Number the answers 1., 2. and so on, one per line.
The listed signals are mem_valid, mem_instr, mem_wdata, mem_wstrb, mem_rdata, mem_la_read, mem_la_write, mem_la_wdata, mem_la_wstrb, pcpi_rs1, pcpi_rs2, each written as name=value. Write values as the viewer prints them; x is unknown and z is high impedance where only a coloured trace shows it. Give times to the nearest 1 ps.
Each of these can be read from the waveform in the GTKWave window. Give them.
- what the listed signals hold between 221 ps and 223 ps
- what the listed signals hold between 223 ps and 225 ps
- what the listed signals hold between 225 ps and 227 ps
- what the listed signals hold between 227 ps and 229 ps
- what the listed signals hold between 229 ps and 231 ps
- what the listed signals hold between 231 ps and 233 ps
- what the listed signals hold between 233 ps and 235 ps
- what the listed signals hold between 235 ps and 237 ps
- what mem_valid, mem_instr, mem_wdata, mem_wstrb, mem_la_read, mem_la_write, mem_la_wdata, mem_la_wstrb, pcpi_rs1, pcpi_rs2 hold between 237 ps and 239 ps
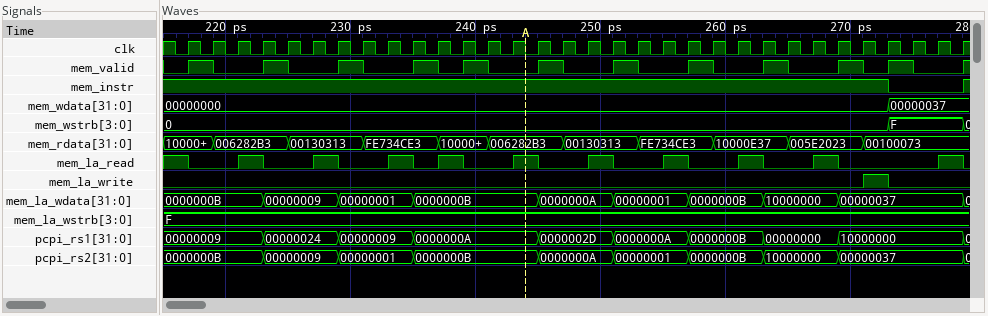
1. mem_valid=0, mem_instr=1, mem_wdata=00000000, mem_wstrb=0, mem_rdata=006282B3, mem_la_read=1, mem_la_write=0, mem_la_wdata=0000000B, mem_la_wstrb=F, pcpi_rs1=00000009, pcpi_rs2=0000000B
2. mem_valid=1, mem_instr=1, mem_wdata=00000000, mem_wstrb=0, mem_rdata=006282B3, mem_la_read=0, mem_la_write=0, mem_la_wdata=00000009, mem_la_wstrb=F, pcpi_rs1=00000024, pcpi_rs2=00000009
3. mem_valid=0, mem_instr=1, mem_wdata=00000000, mem_wstrb=0, mem_rdata=00130313, mem_la_read=0, mem_la_write=0, mem_la_wdata=00000009, mem_la_wstrb=F, pcpi_rs1=00000024, pcpi_rs2=00000009
4. mem_valid=0, mem_instr=1, mem_wdata=00000000, mem_wstrb=0, mem_rdata=00130313, mem_la_read=1, mem_la_write=0, mem_la_wdata=00000009, mem_la_wstrb=F, pcpi_rs1=00000024, pcpi_rs2=00000009
5. mem_valid=1, mem_instr=1, mem_wdata=00000000, mem_wstrb=0, mem_rdata=00130313, mem_la_read=0, mem_la_write=0, mem_la_wdata=00000001, mem_la_wstrb=F, pcpi_rs1=00000009, pcpi_rs2=00000001
6. mem_valid=0, mem_instr=1, mem_wdata=00000000, mem_wstrb=0, mem_rdata=FE734CE3, mem_la_read=0, mem_la_write=0, mem_la_wdata=00000001, mem_la_wstrb=F, pcpi_rs1=00000009, pcpi_rs2=00000001
7. mem_valid=0, mem_instr=1, mem_wdata=00000000, mem_wstrb=0, mem_rdata=FE734CE3, mem_la_read=1, mem_la_write=0, mem_la_wdata=00000001, mem_la_wstrb=F, pcpi_rs1=00000009, pcpi_rs2=00000001
8. mem_valid=1, mem_instr=1, mem_wdata=00000000, mem_wstrb=0, mem_rdata=FE734CE3, mem_la_read=0, mem_la_write=0, mem_la_wdata=0000000B, mem_la_wstrb=F, pcpi_rs1=0000000A, pcpi_rs2=0000000B
9. mem_valid=0, mem_instr=1, mem_wdata=00000000, mem_wstrb=0, mem_la_read=1, mem_la_write=0, mem_la_wdata=0000000B, mem_la_wstrb=F, pcpi_rs1=0000000A, pcpi_rs2=0000000B
